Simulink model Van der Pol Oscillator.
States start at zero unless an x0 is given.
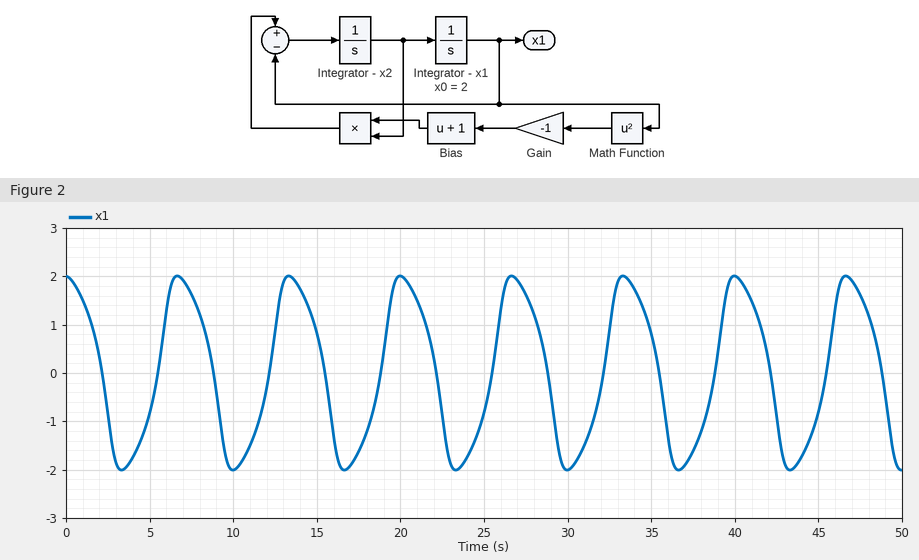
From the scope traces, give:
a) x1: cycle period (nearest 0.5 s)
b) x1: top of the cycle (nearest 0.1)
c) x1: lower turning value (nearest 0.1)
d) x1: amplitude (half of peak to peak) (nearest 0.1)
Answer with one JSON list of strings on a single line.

["6.5 s", "2.0", "-2.0", "2.0"]
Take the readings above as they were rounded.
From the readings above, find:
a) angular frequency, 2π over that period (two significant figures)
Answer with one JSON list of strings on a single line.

["0.97 rad/s"]
